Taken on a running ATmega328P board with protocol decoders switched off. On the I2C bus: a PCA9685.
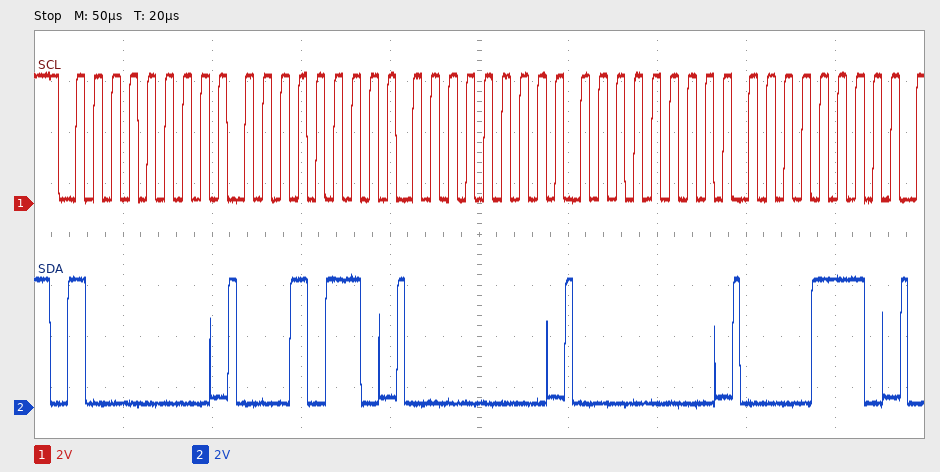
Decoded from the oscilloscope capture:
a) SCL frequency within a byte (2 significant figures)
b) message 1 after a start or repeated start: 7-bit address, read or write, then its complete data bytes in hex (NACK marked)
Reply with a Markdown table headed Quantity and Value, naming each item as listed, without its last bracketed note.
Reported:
| Quantity | Value |
|---|---|
| SCL frequency within a byte | 100 kHz |
| message 1 after a start or repeated start: 7-bit address, read or write, then its complete data bytes in hex | 0x40 write: 16 00 00 0E |
